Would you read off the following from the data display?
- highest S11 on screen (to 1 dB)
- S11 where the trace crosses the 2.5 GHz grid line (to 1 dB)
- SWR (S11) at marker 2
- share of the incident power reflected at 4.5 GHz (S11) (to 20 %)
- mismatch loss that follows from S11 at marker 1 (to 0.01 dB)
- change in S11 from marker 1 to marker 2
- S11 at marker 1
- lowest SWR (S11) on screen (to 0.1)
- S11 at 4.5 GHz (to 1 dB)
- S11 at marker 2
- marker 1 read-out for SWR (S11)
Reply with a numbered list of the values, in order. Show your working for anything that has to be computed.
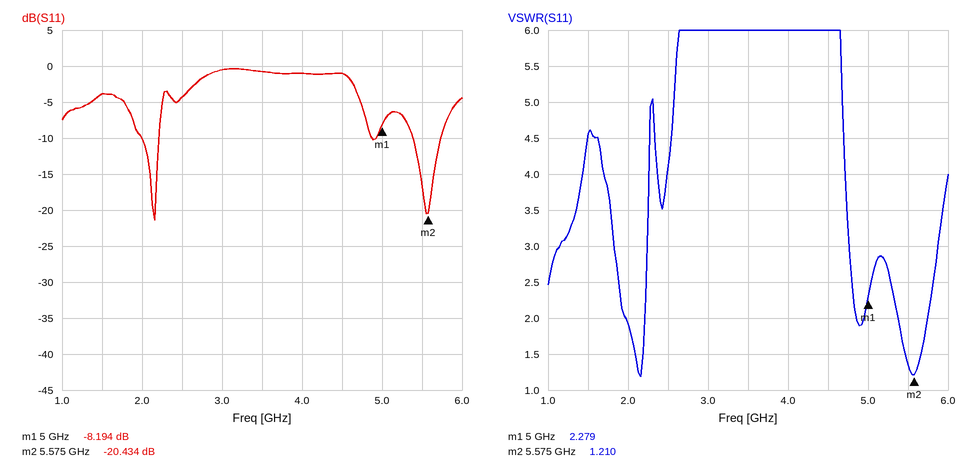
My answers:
1. 0 dB
2. -4 dB
3. 1.210
4. 10^(-1/10) ≈ 79.4 %, so 80 % to the nearest 20 %
5. −10 log10(1 − 10^(-8.194/10)) ≈ 0.71 dB
6. -20.434 − (-8.194) = -12.240 dB
7. -8.194 dB
8. 1.2
9. -1 dB
10. -20.434 dB
11. 2.279
